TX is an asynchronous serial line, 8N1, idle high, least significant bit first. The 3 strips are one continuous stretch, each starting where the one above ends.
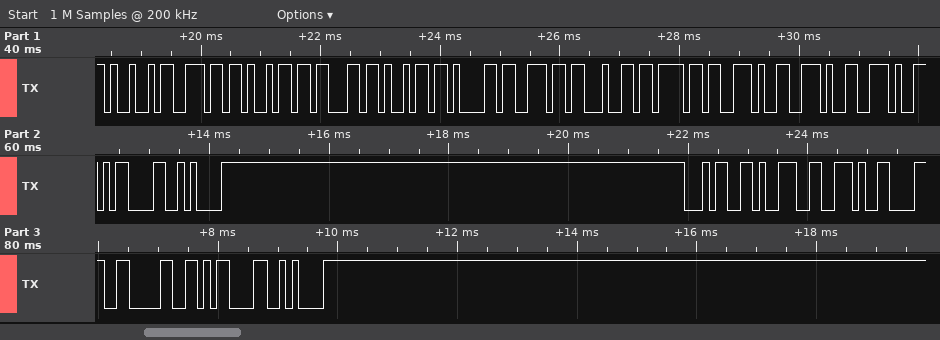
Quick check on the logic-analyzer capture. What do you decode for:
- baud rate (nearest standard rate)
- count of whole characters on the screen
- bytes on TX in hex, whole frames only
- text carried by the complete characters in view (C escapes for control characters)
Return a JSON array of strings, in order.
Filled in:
["9600 baud", "21", "49 6E 69 63 69 61 6E 64 6F 2E 2E 2E 0D 0A 34 39 2E 38 30 0D 0A", "\"Iniciando...\\r\\n49.80\\r\\n\""]
